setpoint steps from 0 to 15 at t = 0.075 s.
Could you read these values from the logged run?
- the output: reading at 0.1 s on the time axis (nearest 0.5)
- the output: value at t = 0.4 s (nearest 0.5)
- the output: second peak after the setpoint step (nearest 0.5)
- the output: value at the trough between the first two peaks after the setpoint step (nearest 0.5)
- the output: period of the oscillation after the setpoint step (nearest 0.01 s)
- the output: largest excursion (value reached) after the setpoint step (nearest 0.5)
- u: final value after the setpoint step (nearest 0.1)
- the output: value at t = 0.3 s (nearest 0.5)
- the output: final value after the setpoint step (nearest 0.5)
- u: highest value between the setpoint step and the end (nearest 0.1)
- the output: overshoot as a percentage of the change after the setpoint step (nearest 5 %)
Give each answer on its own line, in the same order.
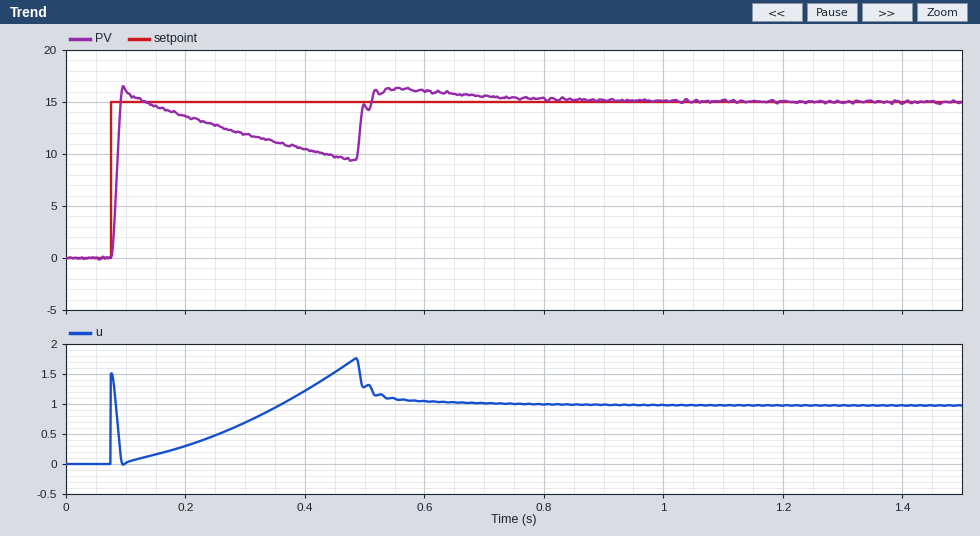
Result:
16.0
10.5
16.5
9.5
0.46 s
16.5
1.0
12.0
15.0
1.8
10 %
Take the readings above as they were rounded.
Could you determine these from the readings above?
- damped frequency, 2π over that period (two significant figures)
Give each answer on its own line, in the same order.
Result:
14 rad/s
